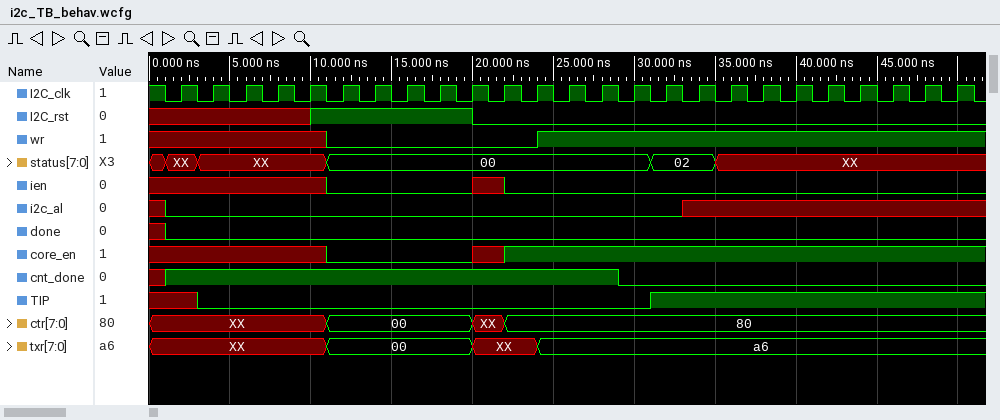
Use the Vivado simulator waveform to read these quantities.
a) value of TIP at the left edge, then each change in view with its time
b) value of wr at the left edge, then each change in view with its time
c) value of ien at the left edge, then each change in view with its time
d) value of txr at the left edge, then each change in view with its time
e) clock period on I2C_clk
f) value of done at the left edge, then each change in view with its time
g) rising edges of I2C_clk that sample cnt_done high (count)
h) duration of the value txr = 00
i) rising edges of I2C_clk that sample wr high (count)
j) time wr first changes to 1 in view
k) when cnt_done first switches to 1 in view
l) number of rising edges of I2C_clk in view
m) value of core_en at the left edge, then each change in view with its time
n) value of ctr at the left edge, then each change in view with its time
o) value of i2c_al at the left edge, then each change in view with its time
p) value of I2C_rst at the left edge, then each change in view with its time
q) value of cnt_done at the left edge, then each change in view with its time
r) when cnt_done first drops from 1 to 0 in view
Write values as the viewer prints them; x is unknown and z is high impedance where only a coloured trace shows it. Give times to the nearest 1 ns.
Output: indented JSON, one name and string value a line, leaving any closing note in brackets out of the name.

{
  "value of TIP at the left edge, then each change in view with its time": "x, 0 at 3 ns, 1 at 31 ns",
  "value of wr at the left edge, then each change in view with its time": "x, 0 at 11 ns, 1 at 24 ns",
  "value of ien at the left edge, then each change in view with its time": "x, 0 at 11 ns, x at 20 ns, 0 at 22 ns",
  "value of txr at the left edge, then each change in view with its time": "XX, 00 at 11 ns, XX at 20 ns, a6 at 24 ns",
  "clock period on I2C_clk": "2 ns",
  "value of done at the left edge, then each change in view with its time": "x, 0 at 1 ns",
  "rising edges of I2C_clk that sample cnt_done high": "14",
  "duration of the value txr = 00": "9 ns",
  "rising edges of I2C_clk that sample wr high": "13",
  "time wr first changes to 1 in view": "24 ns",
  "when cnt_done first switches to 1 in view": "1 ns",
  "number of rising edges of I2C_clk in view": "25",
  "value of core_en at the left edge, then each change in view with its time": "x, 0 at 11 ns, x at 20 ns, 1 at 22 ns",
  "value of ctr at the left edge, then each change in view with its time": "XX, 00 at 11 ns, XX at 20 ns, 80 at 22 ns",
  "value of i2c_al at the left edge, then each change in view with its time": "x, 0 at 1 ns, x at 33 ns",
  "value of I2C_rst at the left edge, then each change in view with its time": "x, 1 at 10 ns, 0 at 20 ns",
  "value of cnt_done at the left edge, then each change in view with its time": "x, 1 at 1 ns, 0 at 29 ns",
  "when cnt_done first drops from 1 to 0 in view": "29 ns"
}
